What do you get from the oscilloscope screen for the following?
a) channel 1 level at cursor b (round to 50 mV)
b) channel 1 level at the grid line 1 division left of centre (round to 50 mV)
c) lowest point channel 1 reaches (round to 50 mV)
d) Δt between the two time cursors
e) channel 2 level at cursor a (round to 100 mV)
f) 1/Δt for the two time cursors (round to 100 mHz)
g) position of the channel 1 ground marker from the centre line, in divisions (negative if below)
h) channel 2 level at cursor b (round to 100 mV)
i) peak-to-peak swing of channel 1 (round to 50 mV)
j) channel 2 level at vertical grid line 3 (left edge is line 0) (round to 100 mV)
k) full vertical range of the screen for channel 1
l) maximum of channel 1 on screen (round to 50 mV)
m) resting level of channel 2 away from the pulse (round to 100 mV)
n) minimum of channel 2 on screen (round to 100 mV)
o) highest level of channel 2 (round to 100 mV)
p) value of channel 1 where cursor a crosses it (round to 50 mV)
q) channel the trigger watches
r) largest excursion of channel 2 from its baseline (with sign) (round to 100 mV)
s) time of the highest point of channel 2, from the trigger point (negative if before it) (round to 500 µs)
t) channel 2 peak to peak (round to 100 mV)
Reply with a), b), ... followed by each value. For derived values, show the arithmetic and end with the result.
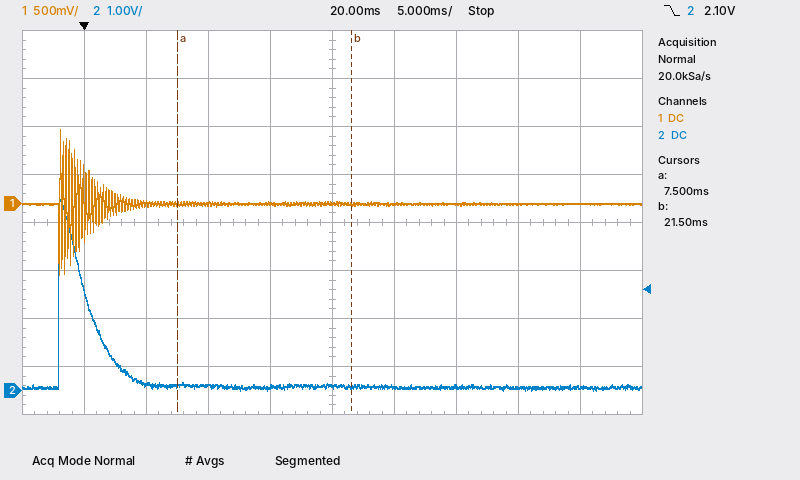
a) 0 mV
b) 0 mV
c) -750 mV
d) 21.5 ms − (7.5 ms) = 14.0 ms
e) 100 mV
f) 1 / 14.0 ms ≈ 71.4 Hz
g) +0.4 div
h) 100 mV
i) 750 mV − (-750 mV) = 1.50 V
j) 100 mV
k) 4 V
l) 750 mV
m) 100 mV
n) 0.0 V
o) 4.0 V
p) 0 mV
q) channel 2
r) 4.0 V − (100 mV) = +3.9 V
s) -2.0 ms
t) 4.0 V − (0.0 V) = 4.0 V
